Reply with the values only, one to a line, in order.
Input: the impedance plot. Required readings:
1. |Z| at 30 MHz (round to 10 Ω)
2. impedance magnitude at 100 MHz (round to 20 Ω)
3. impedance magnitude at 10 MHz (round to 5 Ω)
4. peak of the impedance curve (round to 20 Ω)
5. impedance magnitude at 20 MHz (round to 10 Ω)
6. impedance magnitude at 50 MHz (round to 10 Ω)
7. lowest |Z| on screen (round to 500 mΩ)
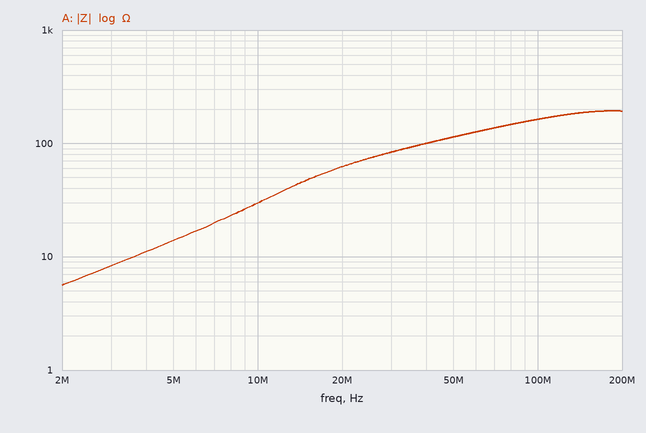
80 Ω
160 Ω
30 Ω
200 Ω
60 Ω
110 Ω
5.5 Ω
